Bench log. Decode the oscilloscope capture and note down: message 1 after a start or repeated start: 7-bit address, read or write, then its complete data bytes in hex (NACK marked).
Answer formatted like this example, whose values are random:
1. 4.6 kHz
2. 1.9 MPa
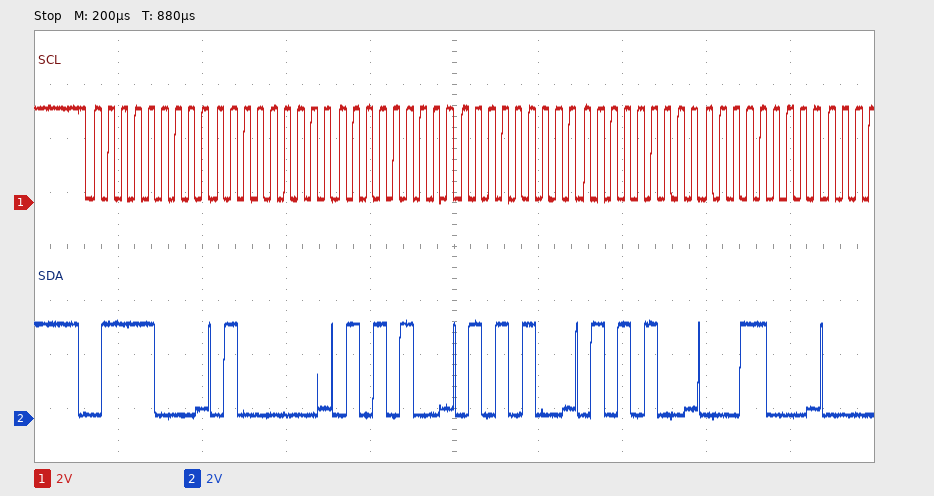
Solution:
1. 0x3C write: 40 54 54 54 18
